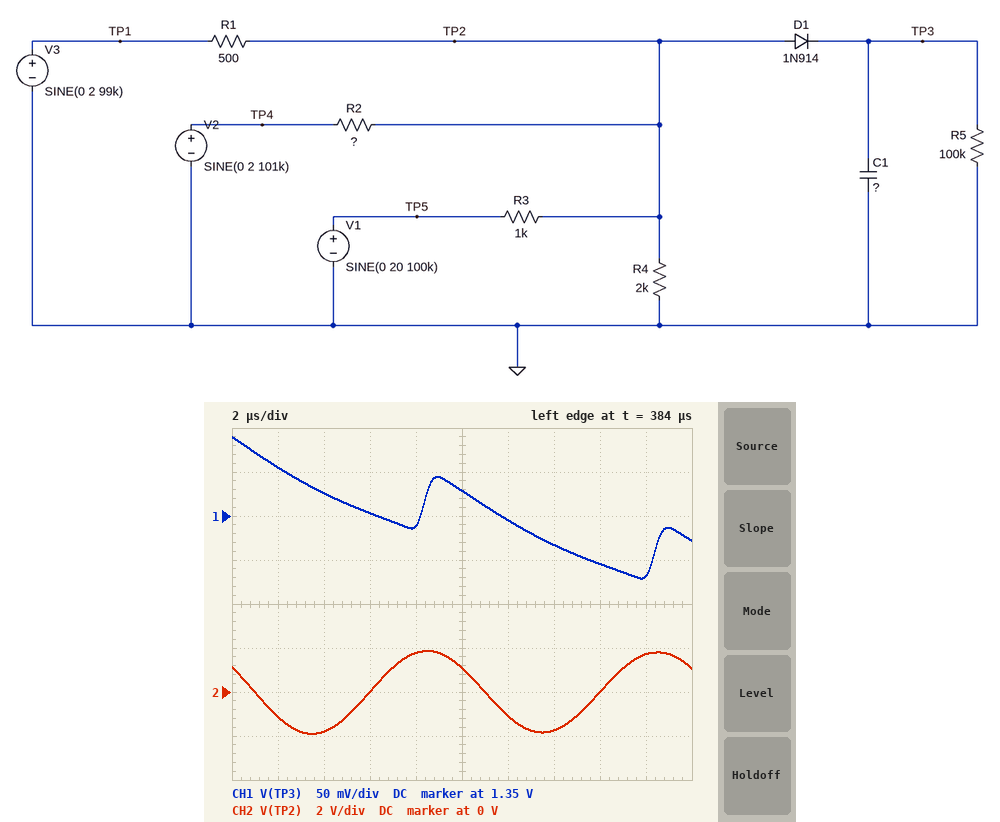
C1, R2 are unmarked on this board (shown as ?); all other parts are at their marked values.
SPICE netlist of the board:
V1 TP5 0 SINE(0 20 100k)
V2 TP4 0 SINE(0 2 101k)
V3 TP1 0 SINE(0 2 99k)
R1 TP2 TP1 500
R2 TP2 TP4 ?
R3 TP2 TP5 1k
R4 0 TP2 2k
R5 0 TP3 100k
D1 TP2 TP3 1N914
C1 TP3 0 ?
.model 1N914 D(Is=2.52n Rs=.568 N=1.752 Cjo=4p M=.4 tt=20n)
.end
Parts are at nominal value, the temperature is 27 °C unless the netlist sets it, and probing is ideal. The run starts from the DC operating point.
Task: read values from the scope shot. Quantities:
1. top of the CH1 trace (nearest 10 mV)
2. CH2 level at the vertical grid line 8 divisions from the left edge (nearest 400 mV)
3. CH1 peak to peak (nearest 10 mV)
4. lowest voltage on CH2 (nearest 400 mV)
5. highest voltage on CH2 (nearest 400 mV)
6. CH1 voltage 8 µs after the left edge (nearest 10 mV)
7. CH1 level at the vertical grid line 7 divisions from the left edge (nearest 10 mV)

1.44 V
0 V
160 mV
-2.0 V
2.0 V
1.34 V
1.32 V
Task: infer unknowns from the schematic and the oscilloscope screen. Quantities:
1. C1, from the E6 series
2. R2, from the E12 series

1 nF
330 Ω
